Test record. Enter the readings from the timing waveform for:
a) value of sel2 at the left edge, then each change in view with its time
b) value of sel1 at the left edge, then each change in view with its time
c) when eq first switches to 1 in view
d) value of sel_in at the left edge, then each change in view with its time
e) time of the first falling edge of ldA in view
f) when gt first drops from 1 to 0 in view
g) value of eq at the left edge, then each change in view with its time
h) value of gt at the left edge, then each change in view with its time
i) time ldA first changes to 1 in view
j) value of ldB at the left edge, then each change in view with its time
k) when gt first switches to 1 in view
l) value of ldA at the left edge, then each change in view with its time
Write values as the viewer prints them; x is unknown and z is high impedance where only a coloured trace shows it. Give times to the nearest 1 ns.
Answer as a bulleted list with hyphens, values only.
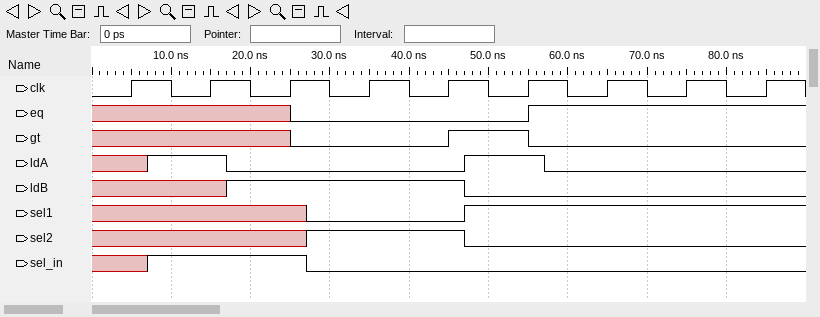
- x, 1 at 27 ns, 0 at 47 ns
- x, 0 at 27 ns, 1 at 47 ns
- 55 ns
- x, 1 at 7 ns, 0 at 27 ns
- 17 ns
- 55 ns
- x, 0 at 25 ns, 1 at 55 ns
- x, 0 at 25 ns, 1 at 45 ns, 0 at 55 ns
- 7 ns
- x, 1 at 17 ns, 0 at 47 ns
- 45 ns
- x, 1 at 7 ns, 0 at 17 ns, 1 at 47 ns, 0 at 57 ns
